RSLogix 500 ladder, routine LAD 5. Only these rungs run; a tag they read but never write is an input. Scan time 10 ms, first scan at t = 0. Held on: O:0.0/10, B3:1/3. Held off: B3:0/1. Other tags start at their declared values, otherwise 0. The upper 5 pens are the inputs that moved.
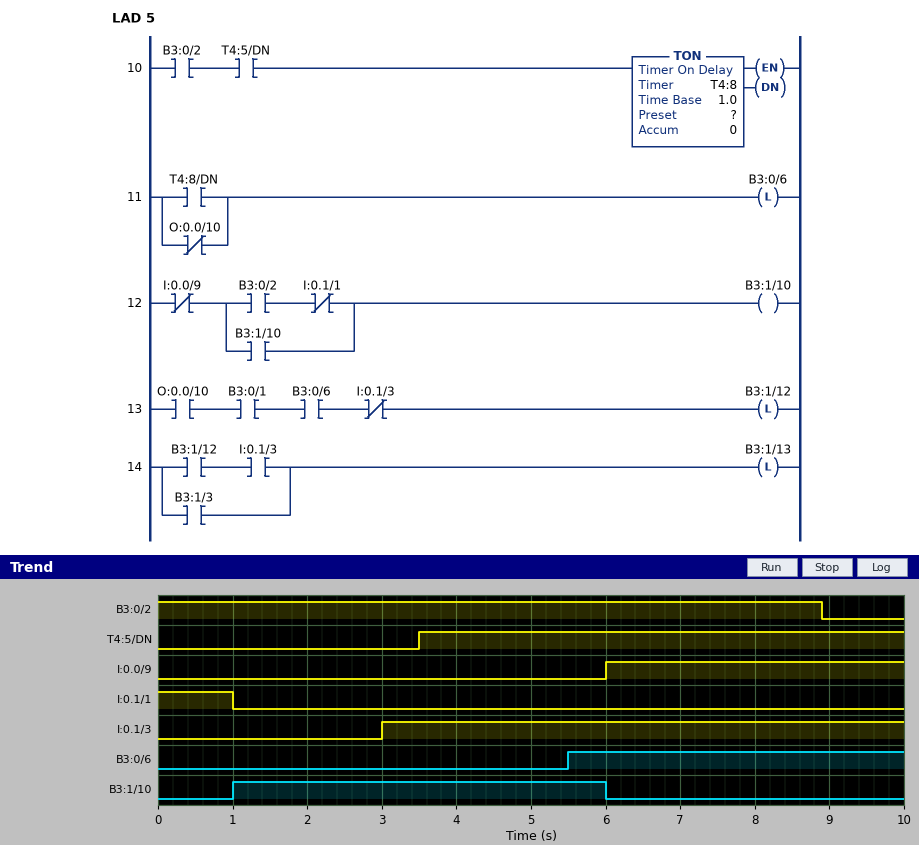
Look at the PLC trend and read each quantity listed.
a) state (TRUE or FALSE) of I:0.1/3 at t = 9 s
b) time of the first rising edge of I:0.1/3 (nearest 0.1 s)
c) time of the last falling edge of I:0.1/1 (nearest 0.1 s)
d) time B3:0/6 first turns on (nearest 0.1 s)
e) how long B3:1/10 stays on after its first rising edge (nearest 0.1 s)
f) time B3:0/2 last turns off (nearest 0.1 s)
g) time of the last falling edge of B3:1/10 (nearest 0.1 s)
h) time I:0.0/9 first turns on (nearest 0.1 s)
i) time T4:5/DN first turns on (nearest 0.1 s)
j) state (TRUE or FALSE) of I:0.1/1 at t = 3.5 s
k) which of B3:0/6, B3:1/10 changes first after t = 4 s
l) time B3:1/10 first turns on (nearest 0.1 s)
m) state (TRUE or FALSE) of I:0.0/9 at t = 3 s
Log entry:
TRUE
3.0 s
1.0 s
5.5 s
5.0 s
8.9 s
6.0 s
6.0 s
3.5 s
FALSE
B3:0/6
1.0 s
FALSE
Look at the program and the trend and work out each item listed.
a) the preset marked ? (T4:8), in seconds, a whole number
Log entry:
2 s
